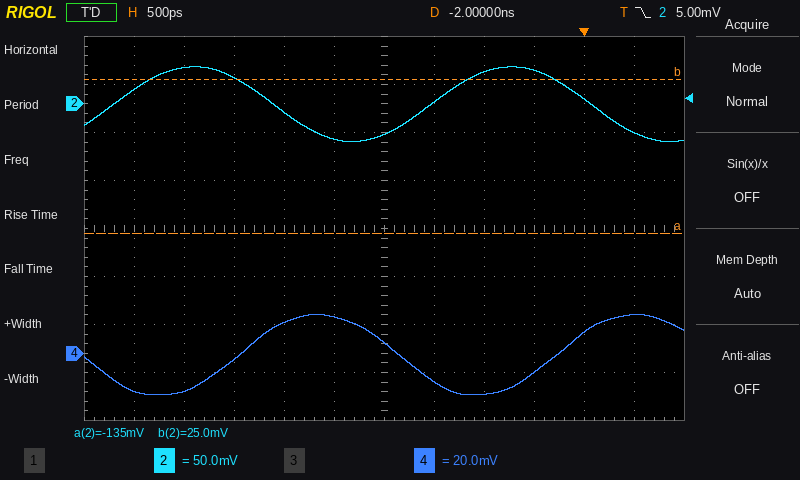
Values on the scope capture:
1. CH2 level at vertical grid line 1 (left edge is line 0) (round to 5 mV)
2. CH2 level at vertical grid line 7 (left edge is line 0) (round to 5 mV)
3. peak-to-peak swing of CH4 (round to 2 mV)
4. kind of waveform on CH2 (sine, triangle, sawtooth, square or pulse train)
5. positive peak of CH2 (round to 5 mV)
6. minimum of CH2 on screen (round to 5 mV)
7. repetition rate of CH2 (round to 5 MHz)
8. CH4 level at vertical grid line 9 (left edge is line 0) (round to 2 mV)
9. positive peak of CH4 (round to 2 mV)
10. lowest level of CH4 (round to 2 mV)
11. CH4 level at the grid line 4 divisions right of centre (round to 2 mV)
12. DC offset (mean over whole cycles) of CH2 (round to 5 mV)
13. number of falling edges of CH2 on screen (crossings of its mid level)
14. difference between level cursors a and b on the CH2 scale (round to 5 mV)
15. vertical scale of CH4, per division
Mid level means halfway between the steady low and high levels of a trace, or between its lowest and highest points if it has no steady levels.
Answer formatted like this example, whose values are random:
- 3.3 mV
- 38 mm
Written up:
- 15 mV
- 0 mV
- 34 mV
- sine
- 40 mV
- -40 mV
- 315 MHz
- -8 mV
- 16 mV
- -18 mV
- 8 mV
- 0 mV
- 2
- 160 mV
- 20 mV
